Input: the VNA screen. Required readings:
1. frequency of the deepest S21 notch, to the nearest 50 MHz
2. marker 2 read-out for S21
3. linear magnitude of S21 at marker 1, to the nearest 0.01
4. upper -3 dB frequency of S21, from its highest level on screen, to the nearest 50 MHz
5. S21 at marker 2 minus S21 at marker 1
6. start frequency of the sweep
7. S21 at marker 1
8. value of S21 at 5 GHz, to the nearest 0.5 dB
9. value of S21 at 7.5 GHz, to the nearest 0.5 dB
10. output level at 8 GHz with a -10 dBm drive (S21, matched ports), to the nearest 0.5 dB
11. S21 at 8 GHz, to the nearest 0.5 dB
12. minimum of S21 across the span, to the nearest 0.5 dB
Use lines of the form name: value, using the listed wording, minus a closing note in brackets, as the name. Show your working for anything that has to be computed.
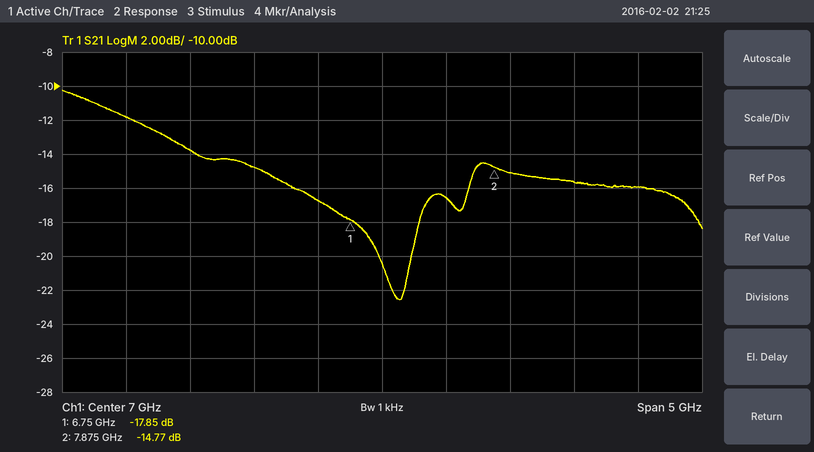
frequency of the deepest S21 notch, to the nearest 50 MHz: 7.15 GHz
marker 2 read-out for S21: -14.77 dB
linear magnitude of S21 at marker 1, to the nearest 0.01: 10^(-17.85/20) ≈ 0.13
upper -3 dB frequency of S21, from its highest level on screen, to the nearest 50 MHz: 5.40 GHz
S21 at marker 2 minus S21 at marker 1: -14.77 − (-17.85) = 3.08 dB
start frequency of the sweep: 4.5 GHz
S21 at marker 1: -17.85 dB
value of S21 at 5 GHz, to the nearest 0.5 dB: -12.0 dB
value of S21 at 7.5 GHz, to the nearest 0.5 dB: -16.5 dB
output level at 8 GHz with a -10 dBm drive (S21, matched ports), to the nearest 0.5 dB: -10 dBm + (-15.0 dB) = -25.0 dBm
S21 at 8 GHz, to the nearest 0.5 dB: -15.0 dB
minimum of S21 across the span, to the nearest 0.5 dB: -22.5 dB
